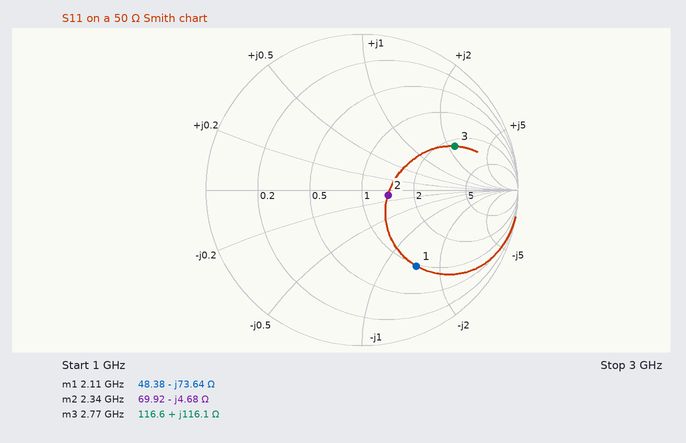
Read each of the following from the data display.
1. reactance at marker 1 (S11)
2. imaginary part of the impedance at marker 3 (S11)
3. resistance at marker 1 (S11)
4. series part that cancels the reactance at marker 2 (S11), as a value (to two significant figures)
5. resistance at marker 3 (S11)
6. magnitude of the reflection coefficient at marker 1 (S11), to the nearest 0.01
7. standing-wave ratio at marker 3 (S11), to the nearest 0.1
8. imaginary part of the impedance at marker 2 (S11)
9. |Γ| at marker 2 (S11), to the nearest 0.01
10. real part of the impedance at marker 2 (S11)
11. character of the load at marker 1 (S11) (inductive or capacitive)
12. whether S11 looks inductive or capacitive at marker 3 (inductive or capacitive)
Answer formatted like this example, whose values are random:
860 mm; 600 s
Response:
-73.64 Ω; +116.1 Ω; 48.38 Ω; 320 pH; 116.6 Ω; 0.60; 4.9; -4.68 Ω; 0.17; 69.92 Ω; capacitive; inductive
